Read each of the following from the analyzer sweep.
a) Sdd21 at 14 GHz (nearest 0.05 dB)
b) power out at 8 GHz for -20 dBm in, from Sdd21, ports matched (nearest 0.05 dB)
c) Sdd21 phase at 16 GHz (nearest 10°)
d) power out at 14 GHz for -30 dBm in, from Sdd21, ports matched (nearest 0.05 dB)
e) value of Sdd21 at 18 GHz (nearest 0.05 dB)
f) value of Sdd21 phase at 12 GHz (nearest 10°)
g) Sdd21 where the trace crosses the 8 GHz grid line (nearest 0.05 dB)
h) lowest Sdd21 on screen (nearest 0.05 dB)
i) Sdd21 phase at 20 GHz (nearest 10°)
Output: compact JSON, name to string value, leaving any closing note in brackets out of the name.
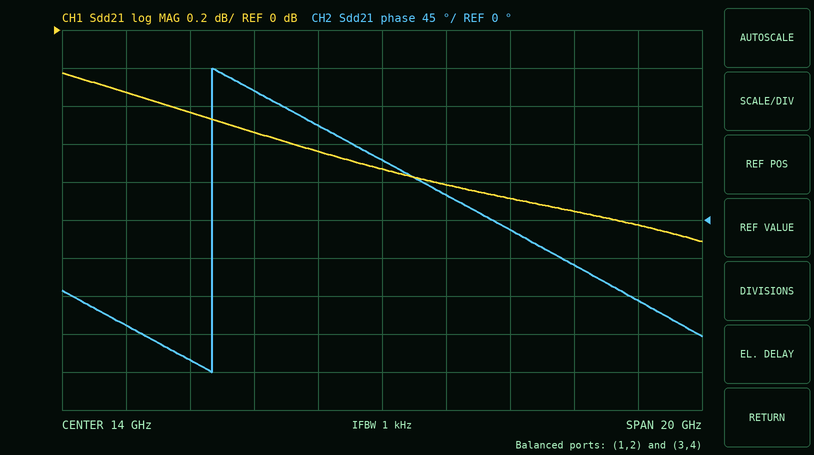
{"Sdd21 at 14 GHz": "-0.75 dB", "power out at 8 GHz for -20 dBm in, from Sdd21, ports matched": "-20.45 dBm", "Sdd21 phase at 16 GHz": "30°", "power out at 14 GHz for -30 dBm in, from Sdd21, ports matched": "-30.75 dBm", "value of Sdd21 at 18 GHz": "-0.90 dB", "value of Sdd21 phase at 12 GHz": "110°", "Sdd21 where the trace crosses the 8 GHz grid line": "-0.45 dB", "lowest Sdd21 on screen": "-1.10 dB", "Sdd21 phase at 20 GHz": "-50°"}
